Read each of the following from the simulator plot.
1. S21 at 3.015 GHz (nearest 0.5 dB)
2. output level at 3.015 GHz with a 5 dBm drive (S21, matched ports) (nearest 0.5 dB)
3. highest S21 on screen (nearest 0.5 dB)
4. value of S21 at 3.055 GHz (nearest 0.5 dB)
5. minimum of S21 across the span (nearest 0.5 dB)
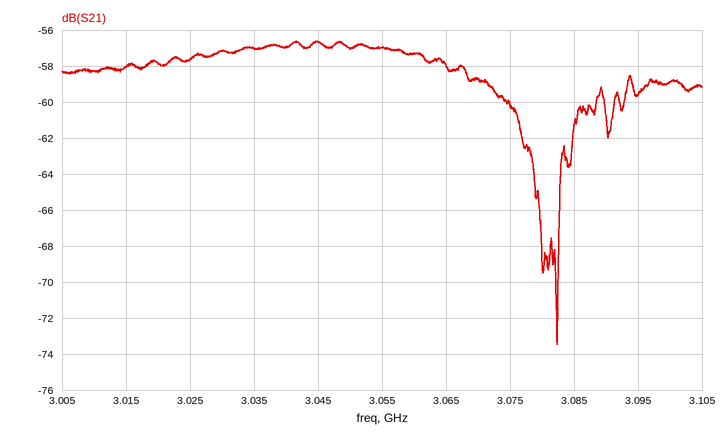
-58.0 dB
-53.0 dBm
-56.5 dB
-57.0 dB
-73.5 dB
